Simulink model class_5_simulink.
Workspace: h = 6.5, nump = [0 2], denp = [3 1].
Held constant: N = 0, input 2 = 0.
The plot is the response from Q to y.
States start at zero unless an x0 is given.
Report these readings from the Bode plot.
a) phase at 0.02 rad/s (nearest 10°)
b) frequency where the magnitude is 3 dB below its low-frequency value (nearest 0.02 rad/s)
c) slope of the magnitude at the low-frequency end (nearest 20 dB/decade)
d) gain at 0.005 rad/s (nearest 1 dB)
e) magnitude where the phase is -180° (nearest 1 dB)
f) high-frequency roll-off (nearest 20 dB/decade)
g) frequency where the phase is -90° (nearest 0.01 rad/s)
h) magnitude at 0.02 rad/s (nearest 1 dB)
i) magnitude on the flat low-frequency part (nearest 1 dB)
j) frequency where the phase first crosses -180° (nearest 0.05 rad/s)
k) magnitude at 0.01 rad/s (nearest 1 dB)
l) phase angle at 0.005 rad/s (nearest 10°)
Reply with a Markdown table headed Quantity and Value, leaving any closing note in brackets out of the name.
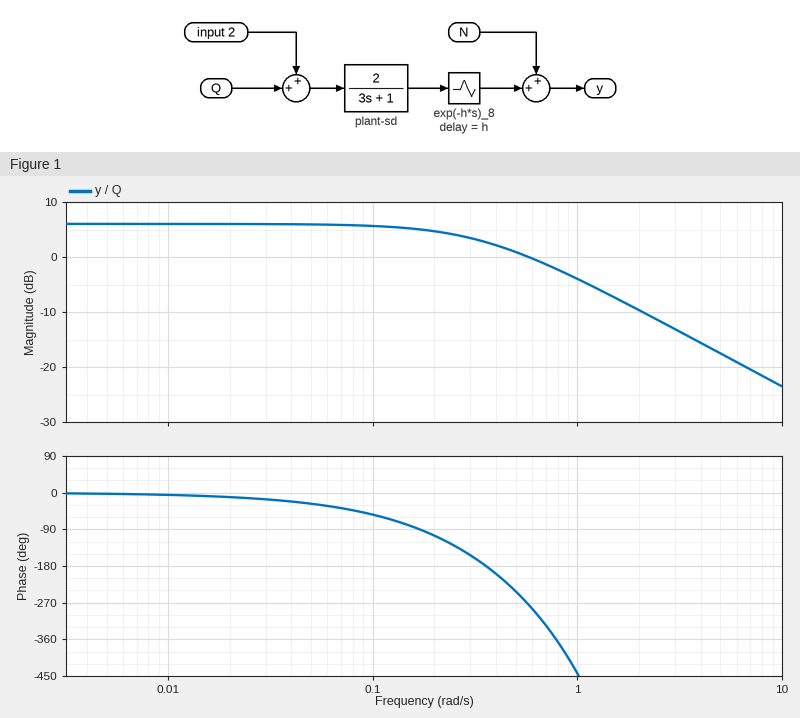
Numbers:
| Quantity | Value |
|---|---|
| phase at 0.02 rad/s | -10° |
| frequency where the magnitude is 3 dB below its low-frequency value | 0.34 rad/s |
| slope of the magnitude at the low-frequency end | 0 dB/decade |
| gain at 0.005 rad/s | 6 dB |
| magnitude where the phase is -180° | 3 dB |
| high-frequency roll-off | -20 dB/decade |
| frequency where the phase is -90° | 0.17 rad/s |
| magnitude at 0.02 rad/s | 6 dB |
| magnitude on the flat low-frequency part | 6 dB |
| frequency where the phase first crosses -180° | 0.35 rad/s |
| magnitude at 0.01 rad/s | 6 dB |
| phase angle at 0.005 rad/s | 0° |
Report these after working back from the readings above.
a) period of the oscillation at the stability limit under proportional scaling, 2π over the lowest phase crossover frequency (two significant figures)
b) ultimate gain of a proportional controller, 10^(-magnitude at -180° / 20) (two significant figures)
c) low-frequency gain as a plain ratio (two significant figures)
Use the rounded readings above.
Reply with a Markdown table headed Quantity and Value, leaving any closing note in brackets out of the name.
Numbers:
| Quantity | Value |
|---|---|
| period of the oscillation at the stability limit under proportional scaling, 2π over the lowest phase crossover frequency | 18 s |
| ultimate gain of a proportional controller, 10^(-magnitude at -180° / 20) | 0.71 |
| low-frequency gain as a plain ratio | 2.0 |
